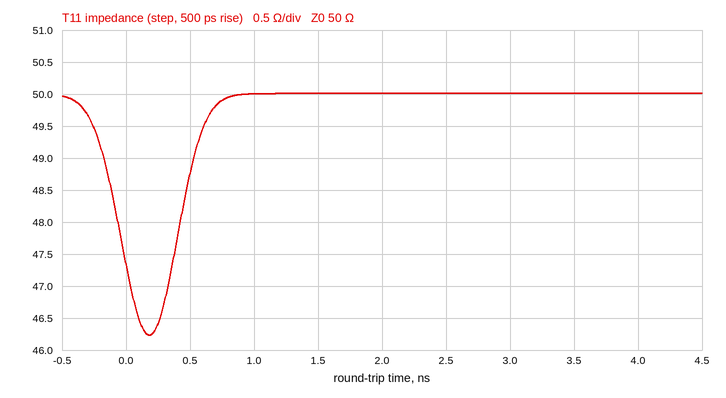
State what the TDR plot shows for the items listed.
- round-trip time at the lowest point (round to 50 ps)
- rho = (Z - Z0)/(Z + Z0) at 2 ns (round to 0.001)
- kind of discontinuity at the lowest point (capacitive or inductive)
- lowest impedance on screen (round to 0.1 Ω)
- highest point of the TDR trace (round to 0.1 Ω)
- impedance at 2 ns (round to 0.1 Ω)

200 ps
0.000
capacitive
46.2 Ω
50.0 Ω
50.0 Ω
